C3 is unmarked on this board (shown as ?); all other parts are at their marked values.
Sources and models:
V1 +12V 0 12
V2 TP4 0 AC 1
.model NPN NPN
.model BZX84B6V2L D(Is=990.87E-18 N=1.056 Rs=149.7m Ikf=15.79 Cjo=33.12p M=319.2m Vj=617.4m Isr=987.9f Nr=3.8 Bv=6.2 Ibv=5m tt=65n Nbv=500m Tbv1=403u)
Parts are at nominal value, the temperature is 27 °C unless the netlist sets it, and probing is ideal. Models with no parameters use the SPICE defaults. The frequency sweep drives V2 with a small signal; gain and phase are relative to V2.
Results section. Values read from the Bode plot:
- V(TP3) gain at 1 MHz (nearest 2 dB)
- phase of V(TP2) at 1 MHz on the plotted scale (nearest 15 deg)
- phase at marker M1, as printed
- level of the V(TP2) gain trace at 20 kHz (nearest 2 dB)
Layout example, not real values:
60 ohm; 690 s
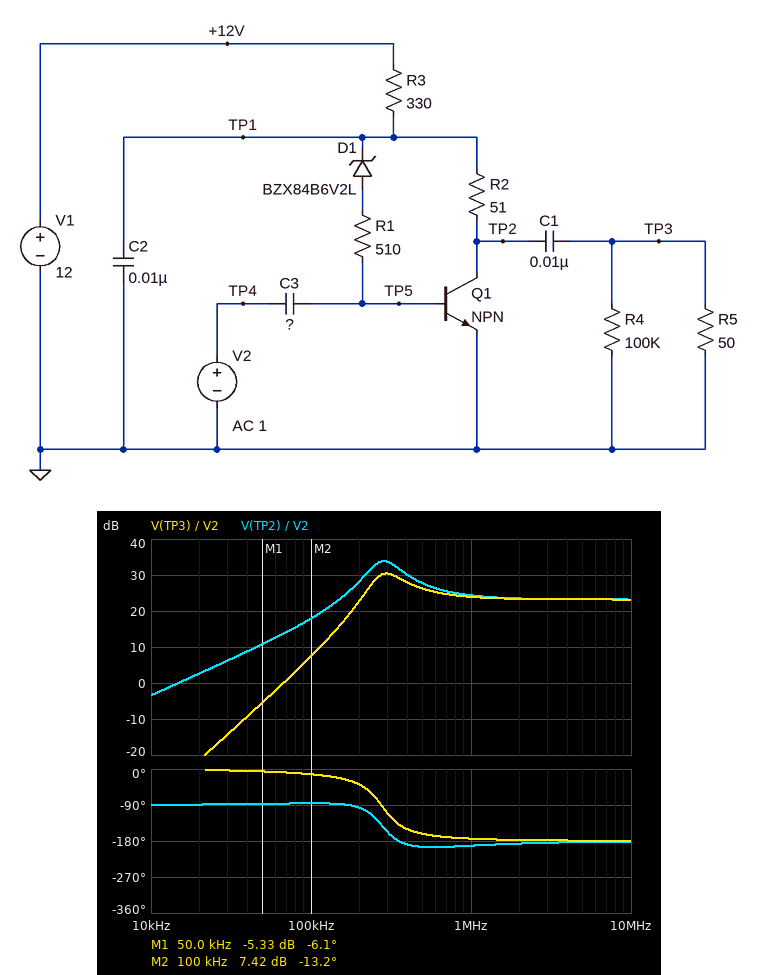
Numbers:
24 dB; -195 deg; -6.1 deg; 2 dB
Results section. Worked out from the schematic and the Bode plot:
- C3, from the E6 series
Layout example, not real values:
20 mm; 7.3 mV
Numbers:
15 nF
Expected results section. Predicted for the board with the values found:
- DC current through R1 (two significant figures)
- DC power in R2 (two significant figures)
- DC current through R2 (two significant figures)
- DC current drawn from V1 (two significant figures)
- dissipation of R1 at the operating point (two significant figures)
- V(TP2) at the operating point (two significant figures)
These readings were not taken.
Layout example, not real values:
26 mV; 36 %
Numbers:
150 µA; 11 mW; 15 mA; 15 mA; 11 µW; 6.3 V
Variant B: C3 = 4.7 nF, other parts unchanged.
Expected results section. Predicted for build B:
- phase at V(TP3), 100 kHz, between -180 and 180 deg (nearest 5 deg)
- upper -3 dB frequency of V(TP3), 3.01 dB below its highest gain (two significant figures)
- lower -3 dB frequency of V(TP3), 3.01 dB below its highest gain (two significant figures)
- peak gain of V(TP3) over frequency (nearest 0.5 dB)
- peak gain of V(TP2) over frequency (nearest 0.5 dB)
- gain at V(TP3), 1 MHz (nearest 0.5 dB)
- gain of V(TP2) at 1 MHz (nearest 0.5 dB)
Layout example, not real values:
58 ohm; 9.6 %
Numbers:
-10 deg; 1.1 MHz; 430 kHz; 28.0 dB; 29.0 dB; 25.0 dB; 25.5 dB
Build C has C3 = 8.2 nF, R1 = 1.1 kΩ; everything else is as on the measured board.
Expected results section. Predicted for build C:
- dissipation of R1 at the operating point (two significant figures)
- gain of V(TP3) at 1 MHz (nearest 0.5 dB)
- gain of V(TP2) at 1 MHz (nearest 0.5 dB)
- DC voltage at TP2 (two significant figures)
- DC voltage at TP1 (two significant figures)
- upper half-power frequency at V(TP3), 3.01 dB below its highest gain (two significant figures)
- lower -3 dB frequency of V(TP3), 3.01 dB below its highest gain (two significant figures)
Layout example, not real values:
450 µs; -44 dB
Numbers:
23 µW; 23.5 dB; 24.0 dB; 6.4 V; 7.2 V; 560 kHz; 230 kHz
